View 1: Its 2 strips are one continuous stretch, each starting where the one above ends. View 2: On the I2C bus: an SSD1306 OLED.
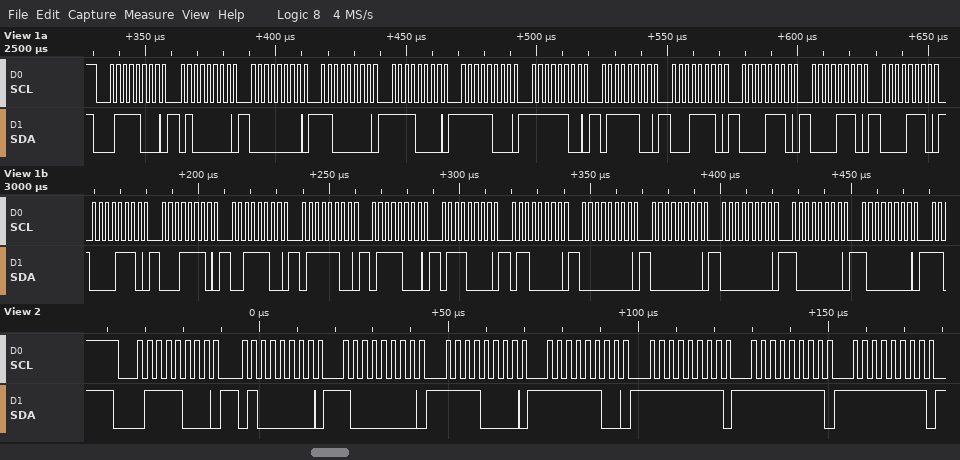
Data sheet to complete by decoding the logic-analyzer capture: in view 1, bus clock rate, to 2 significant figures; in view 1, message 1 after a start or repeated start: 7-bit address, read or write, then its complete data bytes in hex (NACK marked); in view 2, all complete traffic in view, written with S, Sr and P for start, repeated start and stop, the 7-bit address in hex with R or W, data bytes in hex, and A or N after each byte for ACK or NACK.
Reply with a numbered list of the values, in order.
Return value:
1. 400 kHz
2. 0x3C write: 40 00 C0 F0 F8 FC 7C 1E 0E 0E 0E 0E 1E 3C 7C 78 70 60 00 00 00 80 80
3. S 3CW A 40 A 80 A F0 A FC A FF A FF A FF A
